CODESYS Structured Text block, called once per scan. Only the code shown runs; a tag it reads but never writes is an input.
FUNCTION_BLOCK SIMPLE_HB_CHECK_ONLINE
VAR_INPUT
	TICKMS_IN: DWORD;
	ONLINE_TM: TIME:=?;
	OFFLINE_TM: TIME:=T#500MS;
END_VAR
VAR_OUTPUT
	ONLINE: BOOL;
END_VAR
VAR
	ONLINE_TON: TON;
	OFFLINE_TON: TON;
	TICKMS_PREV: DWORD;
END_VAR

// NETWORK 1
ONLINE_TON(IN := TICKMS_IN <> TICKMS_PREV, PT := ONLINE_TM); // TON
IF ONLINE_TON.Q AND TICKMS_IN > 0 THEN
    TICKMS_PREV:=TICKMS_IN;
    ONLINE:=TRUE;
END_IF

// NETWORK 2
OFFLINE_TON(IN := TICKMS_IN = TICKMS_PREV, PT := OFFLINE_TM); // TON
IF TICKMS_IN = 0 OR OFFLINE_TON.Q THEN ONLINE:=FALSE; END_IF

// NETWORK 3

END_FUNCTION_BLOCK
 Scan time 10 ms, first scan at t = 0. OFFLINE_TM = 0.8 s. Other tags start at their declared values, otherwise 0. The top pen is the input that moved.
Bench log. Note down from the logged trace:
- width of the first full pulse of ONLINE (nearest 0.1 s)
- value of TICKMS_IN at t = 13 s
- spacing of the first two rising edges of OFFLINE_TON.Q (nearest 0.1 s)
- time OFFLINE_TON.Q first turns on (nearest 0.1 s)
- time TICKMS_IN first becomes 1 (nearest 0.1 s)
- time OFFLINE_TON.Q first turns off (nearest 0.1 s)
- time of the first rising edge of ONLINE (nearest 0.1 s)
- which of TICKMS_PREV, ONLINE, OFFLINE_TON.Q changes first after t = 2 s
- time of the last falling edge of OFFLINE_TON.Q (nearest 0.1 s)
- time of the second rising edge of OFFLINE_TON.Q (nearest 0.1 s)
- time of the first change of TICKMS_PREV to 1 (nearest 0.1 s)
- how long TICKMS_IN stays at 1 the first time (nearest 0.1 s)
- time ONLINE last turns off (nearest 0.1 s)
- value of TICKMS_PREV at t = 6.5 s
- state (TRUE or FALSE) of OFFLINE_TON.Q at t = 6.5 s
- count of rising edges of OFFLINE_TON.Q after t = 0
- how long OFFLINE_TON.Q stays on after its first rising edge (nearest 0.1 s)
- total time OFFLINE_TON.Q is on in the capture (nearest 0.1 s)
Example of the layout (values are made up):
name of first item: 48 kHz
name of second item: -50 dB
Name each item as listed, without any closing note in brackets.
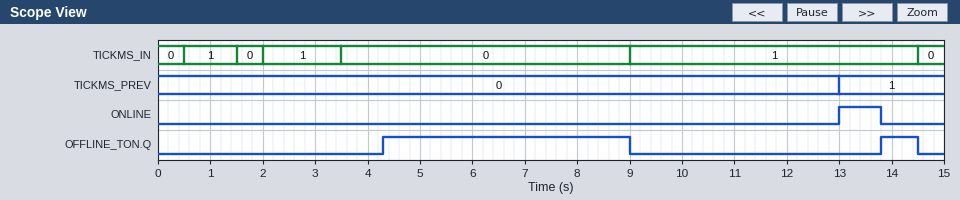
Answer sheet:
width of the first full pulse of ONLINE: 0.8 s
value of TICKMS_IN at t = 13 s: 1
spacing of the first two rising edges of OFFLINE_TON.Q: 9.5 s
time OFFLINE_TON.Q first turns on: 4.3 s
time TICKMS_IN first becomes 1: 0.5 s
time OFFLINE_TON.Q first turns off: 9.0 s
time of the first rising edge of ONLINE: 13.0 s
which of TICKMS_PREV, ONLINE, OFFLINE_TON.Q changes first after t = 2 s: OFFLINE_TON.Q
time of the last falling edge of OFFLINE_TON.Q: 14.5 s
time of the second rising edge of OFFLINE_TON.Q: 13.8 s
time of the first change of TICKMS_PREV to 1: 13.0 s
how long TICKMS_IN stays at 1 the first time: 1.0 s
time ONLINE last turns off: 13.8 s
value of TICKMS_PREV at t = 6.5 s: 0
state (TRUE or FALSE) of OFFLINE_TON.Q at t = 6.5 s: TRUE
count of rising edges of OFFLINE_TON.Q after t = 0: 2
how long OFFLINE_TON.Q stays on after its first rising edge: 4.7 s
total time OFFLINE_TON.Q is on in the capture: 5.4 s
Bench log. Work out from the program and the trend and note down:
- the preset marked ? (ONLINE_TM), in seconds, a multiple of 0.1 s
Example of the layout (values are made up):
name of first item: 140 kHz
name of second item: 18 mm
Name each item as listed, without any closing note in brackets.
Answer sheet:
the preset marked ? (ONLINE_TM), in seconds, a multiple of 0.1 s: 4.0 s
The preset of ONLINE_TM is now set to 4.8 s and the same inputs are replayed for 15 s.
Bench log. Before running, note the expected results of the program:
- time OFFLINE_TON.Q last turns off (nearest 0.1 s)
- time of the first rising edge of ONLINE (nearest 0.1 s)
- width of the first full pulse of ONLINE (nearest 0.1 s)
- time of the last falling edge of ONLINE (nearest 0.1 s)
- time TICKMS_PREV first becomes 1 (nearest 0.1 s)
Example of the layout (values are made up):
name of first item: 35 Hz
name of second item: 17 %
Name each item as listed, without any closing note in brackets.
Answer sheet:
time OFFLINE_TON.Q last turns off: 9.0 s
time of the first rising edge of ONLINE: 13.8 s
width of the first full pulse of ONLINE: 0.7 s
time of the last falling edge of ONLINE: 14.5 s
time TICKMS_PREV first becomes 1: 13.8 s
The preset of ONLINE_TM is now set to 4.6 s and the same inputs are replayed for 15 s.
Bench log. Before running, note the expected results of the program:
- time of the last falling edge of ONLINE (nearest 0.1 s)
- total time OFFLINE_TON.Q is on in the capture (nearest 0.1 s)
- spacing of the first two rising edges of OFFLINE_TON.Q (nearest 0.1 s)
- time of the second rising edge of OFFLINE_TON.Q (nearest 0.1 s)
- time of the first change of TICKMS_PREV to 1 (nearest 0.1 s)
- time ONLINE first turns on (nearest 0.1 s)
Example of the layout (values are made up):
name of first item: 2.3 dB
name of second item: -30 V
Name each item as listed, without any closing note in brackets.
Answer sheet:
time of the last falling edge of ONLINE: 14.4 s
total time OFFLINE_TON.Q is on in the capture: 4.8 s
spacing of the first two rising edges of OFFLINE_TON.Q: 10.1 s
time of the second rising edge of OFFLINE_TON.Q: 14.4 s
time of the first change of TICKMS_PREV to 1: 13.6 s
time ONLINE first turns on: 13.6 s
